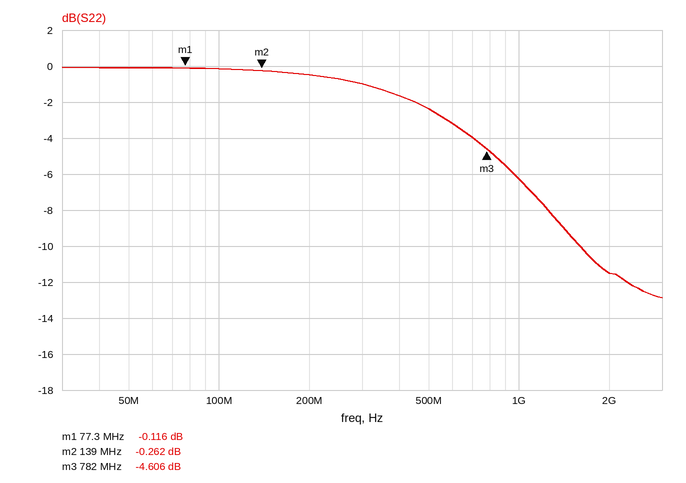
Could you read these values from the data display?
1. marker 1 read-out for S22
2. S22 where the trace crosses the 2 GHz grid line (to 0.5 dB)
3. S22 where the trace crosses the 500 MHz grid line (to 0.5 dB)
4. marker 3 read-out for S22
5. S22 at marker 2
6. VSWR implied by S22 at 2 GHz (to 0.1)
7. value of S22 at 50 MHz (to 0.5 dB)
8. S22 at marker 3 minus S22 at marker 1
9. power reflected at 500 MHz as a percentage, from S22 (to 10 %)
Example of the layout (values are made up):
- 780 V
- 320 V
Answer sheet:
- -0.116 dB
- -11.5 dB
- -2.5 dB
- -4.606 dB
- -0.262 dB
- 1.7
- 0.0 dB
- -4.490 dB
- 60 %
